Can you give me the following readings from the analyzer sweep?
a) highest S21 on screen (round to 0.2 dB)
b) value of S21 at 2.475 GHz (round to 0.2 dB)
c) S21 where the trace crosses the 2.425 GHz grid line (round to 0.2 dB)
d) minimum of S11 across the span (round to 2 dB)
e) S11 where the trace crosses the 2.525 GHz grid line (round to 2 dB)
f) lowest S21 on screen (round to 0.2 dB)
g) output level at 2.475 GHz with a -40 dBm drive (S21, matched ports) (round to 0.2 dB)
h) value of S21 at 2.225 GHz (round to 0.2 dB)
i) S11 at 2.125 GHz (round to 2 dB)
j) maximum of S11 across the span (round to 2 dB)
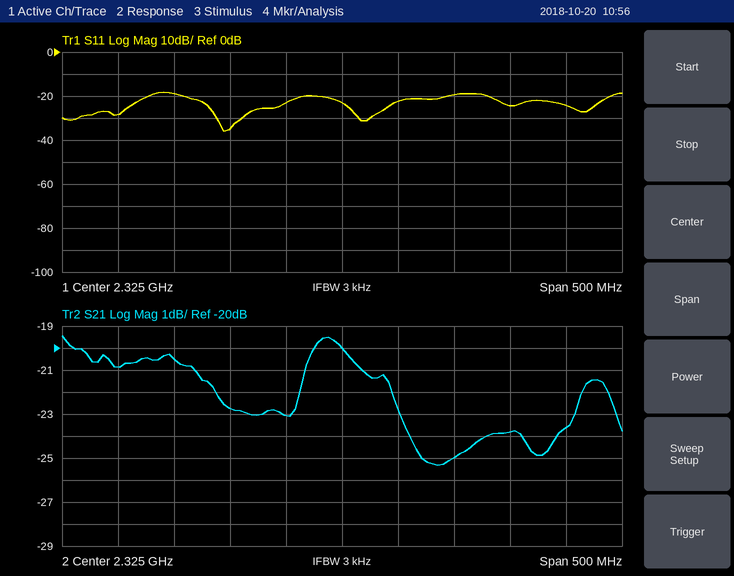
-19.4 dB
-23.8 dB
-25.0 dB
-36 dB
-24 dB
-25.4 dB
-63.8 dBm
-22.8 dB
-28 dB
-18 dB
